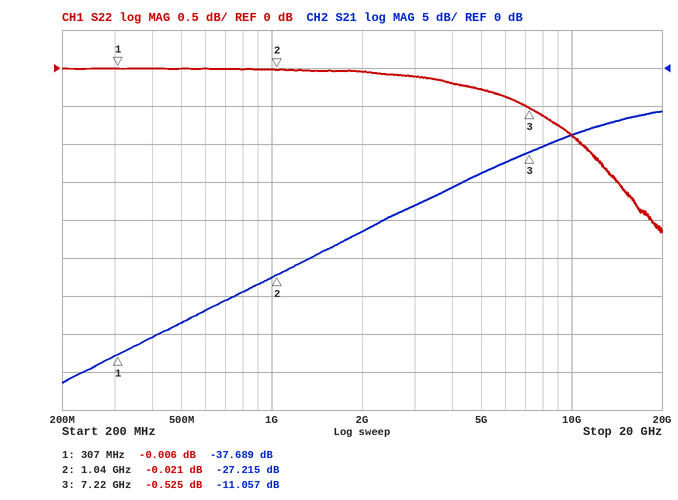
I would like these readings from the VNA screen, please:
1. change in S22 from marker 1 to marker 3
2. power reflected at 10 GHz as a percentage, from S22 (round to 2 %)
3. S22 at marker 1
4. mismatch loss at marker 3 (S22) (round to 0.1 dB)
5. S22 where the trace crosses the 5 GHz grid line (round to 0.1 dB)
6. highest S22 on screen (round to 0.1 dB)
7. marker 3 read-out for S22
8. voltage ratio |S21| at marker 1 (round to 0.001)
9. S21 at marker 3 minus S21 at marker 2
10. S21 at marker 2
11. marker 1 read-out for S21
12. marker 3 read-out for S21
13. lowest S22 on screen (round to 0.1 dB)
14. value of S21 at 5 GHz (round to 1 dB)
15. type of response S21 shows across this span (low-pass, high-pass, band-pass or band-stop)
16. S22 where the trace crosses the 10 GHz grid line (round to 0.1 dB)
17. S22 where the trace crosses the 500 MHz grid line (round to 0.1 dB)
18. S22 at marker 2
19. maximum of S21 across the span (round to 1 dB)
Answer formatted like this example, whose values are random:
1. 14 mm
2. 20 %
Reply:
1. -0.519 dB
2. 82 %
3. -0.006 dB
4. 9.4 dB
5. -0.3 dB
6. 0.0 dB
7. -0.525 dB
8. 0.013
9. 16.158 dB
10. -27.215 dB
11. -37.689 dB
12. -11.057 dB
13. -2.2 dB
14. -14 dB
15. high-pass
16. -0.9 dB
17. 0.0 dB
18. -0.021 dB
19. -6 dB
